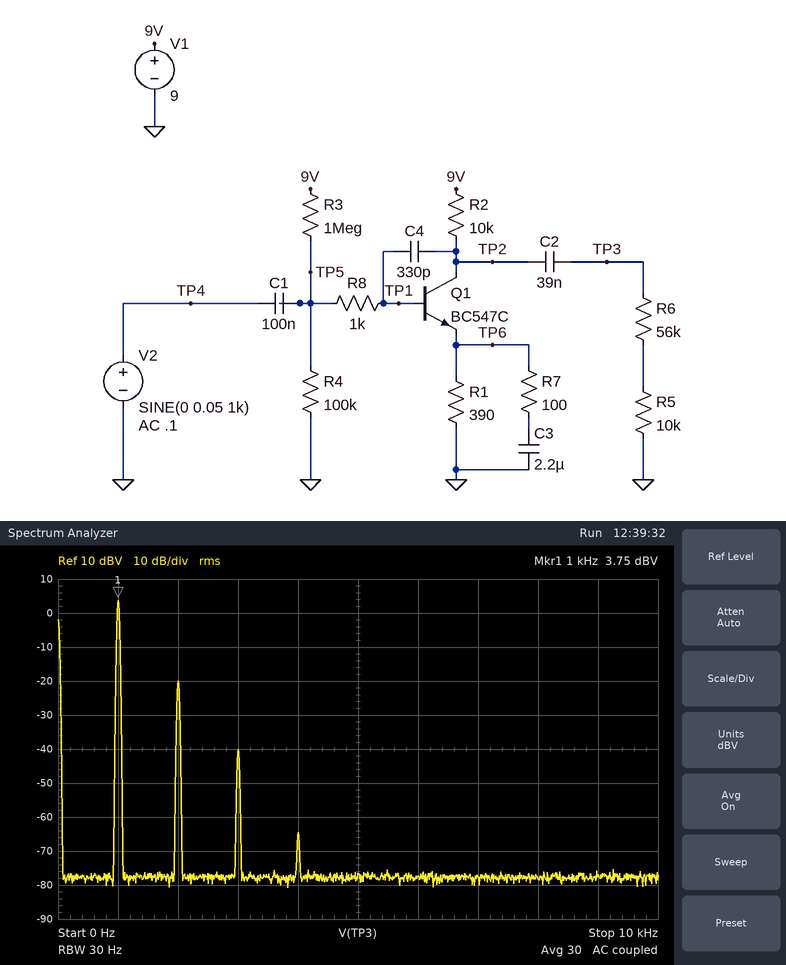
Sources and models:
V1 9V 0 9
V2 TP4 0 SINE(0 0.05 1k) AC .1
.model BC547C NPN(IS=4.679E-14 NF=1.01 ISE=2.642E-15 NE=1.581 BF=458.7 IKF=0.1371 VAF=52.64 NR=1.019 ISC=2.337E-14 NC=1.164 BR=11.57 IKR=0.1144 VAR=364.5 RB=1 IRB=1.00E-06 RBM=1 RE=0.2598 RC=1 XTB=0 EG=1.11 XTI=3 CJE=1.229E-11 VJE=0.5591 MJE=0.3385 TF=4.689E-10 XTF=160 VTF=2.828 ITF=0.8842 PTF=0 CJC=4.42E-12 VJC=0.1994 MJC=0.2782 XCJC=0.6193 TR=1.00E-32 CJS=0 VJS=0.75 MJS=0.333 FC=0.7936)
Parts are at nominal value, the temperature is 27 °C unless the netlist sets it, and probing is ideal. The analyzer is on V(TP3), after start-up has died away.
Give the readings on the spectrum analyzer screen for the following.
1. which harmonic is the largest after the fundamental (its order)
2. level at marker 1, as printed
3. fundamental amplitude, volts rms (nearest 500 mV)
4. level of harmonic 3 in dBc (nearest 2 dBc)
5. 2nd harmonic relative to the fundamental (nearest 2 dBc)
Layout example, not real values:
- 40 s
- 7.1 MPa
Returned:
- 2
- 3.75 dBV
- 1.5 V
- -44 dBc
- -24 dBc
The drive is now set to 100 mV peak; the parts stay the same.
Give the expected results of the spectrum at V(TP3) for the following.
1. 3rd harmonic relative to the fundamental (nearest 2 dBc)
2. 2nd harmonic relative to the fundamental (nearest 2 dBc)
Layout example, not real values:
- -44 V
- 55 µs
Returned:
- -32 dBc
- -16 dBc
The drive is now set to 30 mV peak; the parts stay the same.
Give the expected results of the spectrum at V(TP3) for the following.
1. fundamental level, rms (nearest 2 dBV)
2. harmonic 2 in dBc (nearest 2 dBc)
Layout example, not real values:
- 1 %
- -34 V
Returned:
- 0 dBV
- -28 dBc
